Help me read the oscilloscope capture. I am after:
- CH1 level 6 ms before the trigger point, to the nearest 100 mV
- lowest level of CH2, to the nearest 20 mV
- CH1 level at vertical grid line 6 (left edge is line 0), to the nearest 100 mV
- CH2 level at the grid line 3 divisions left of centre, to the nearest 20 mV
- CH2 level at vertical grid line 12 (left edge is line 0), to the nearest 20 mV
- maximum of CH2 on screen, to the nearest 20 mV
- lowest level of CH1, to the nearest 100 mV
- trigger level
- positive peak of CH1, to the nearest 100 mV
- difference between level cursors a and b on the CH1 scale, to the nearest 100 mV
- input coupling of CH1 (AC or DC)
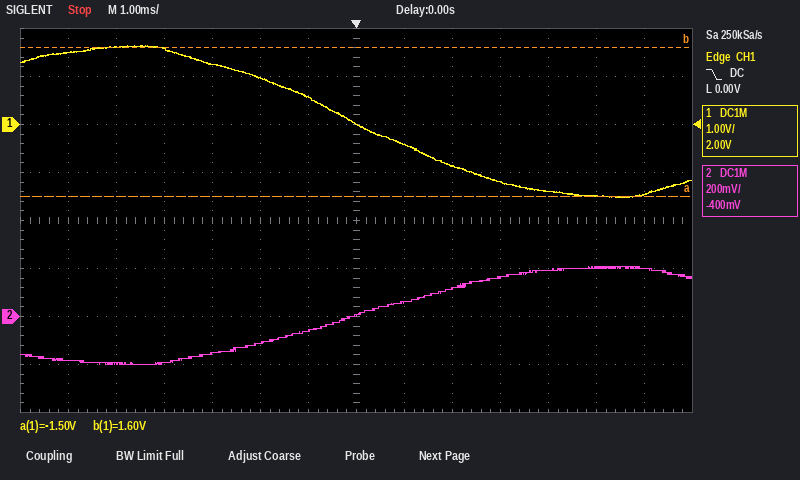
1.5 V
-200 mV
600 mV
-160 mV
200 mV
200 mV
-1.5 V
0.00 V
1.6 V
3.1 V
DC
